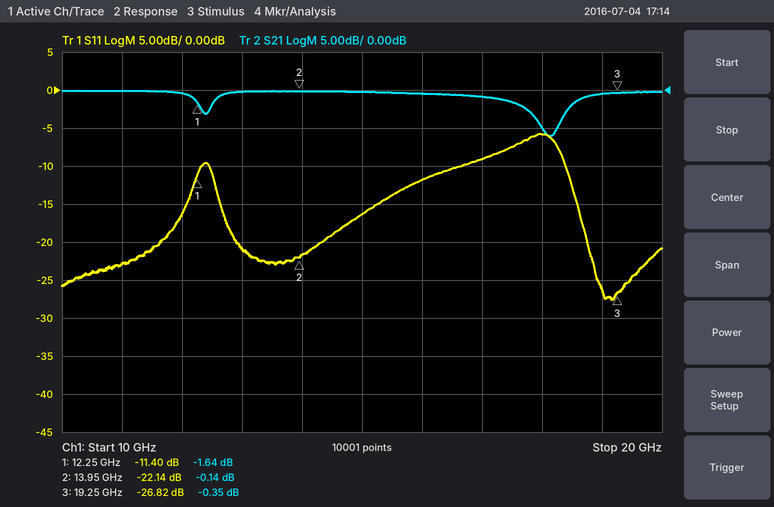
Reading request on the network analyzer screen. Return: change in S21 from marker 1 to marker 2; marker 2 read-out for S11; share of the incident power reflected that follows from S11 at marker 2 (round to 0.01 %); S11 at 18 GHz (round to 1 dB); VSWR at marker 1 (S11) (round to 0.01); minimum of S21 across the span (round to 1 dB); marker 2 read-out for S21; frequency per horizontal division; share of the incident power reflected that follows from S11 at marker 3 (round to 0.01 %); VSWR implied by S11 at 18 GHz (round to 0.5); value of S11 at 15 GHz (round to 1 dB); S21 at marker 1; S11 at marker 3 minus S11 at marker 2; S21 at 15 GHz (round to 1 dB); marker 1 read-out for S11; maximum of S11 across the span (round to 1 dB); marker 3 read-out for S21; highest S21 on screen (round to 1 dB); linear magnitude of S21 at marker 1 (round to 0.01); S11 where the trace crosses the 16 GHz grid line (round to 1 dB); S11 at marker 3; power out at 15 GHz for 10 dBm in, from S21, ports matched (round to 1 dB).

1.50 dB
-22.14 dB
0.61 %
-6 dB
1.74
-6 dB
-0.14 dB
1 GHz
0.21 %
3.0
-16 dB
-1.64 dB
-4.68 dB
0 dB
-11.40 dB
-6 dB
-0.35 dB
0 dB
0.83
-12 dB
-26.82 dB
10 dBm
